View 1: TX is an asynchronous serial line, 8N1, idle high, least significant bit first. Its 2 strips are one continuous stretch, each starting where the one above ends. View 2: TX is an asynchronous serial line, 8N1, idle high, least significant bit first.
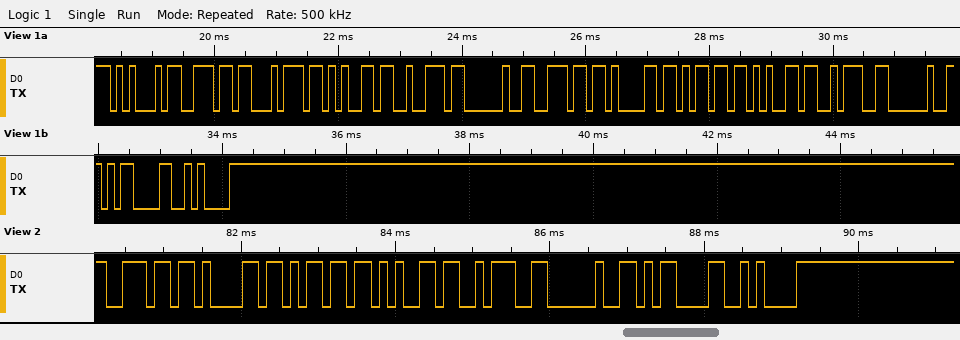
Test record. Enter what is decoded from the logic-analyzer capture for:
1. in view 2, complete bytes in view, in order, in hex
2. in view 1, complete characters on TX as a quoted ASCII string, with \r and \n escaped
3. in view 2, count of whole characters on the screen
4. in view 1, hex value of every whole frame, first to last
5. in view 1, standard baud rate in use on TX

6E 61 6D 65 3A 20 0D 0A
"Enter name: \r\n"
8
45 6E 74 65 72 20 6E 61 6D 65 3A 20 0D 0A
9600 baud
